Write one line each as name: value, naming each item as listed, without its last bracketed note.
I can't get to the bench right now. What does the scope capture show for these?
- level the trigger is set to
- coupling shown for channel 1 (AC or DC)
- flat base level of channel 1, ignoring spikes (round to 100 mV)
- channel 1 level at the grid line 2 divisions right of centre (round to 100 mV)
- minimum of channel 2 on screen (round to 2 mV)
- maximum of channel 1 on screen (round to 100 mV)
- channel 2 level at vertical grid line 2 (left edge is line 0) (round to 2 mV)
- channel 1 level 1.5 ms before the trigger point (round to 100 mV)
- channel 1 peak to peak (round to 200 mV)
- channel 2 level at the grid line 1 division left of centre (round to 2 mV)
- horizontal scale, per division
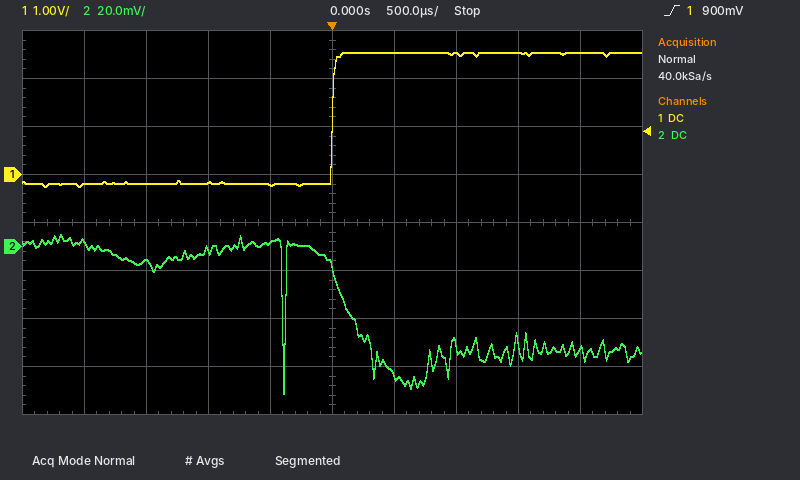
level the trigger is set to: 900 mV
coupling shown for channel 1: DC
flat base level of channel 1, ignoring spikes: -200 mV
channel 1 level at the grid line 2 divisions right of centre: 2.5 V
minimum of channel 2 on screen: -62 mV
maximum of channel 1 on screen: 2.5 V
channel 2 level at vertical grid line 2 (left edge is line 0): -6 mV
channel 1 level 1.5 ms before the trigger point: -200 mV
channel 1 peak to peak: 2.8 V
channel 2 level at the grid line 1 division left of centre: 2 mV
horizontal scale, per division: 500 µs
